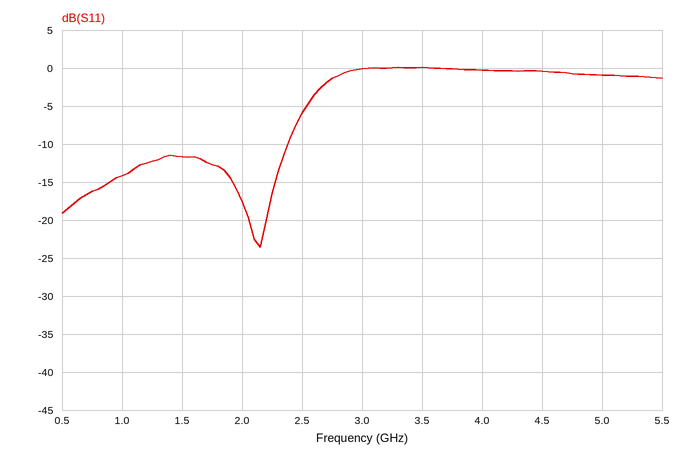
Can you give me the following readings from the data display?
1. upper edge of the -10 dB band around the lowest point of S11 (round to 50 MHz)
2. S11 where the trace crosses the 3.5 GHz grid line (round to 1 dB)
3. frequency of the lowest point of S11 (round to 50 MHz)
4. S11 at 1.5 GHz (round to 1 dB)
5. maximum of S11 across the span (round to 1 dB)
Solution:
2.40 GHz
0 dB
2.15 GHz
-12 dB
0 dB
